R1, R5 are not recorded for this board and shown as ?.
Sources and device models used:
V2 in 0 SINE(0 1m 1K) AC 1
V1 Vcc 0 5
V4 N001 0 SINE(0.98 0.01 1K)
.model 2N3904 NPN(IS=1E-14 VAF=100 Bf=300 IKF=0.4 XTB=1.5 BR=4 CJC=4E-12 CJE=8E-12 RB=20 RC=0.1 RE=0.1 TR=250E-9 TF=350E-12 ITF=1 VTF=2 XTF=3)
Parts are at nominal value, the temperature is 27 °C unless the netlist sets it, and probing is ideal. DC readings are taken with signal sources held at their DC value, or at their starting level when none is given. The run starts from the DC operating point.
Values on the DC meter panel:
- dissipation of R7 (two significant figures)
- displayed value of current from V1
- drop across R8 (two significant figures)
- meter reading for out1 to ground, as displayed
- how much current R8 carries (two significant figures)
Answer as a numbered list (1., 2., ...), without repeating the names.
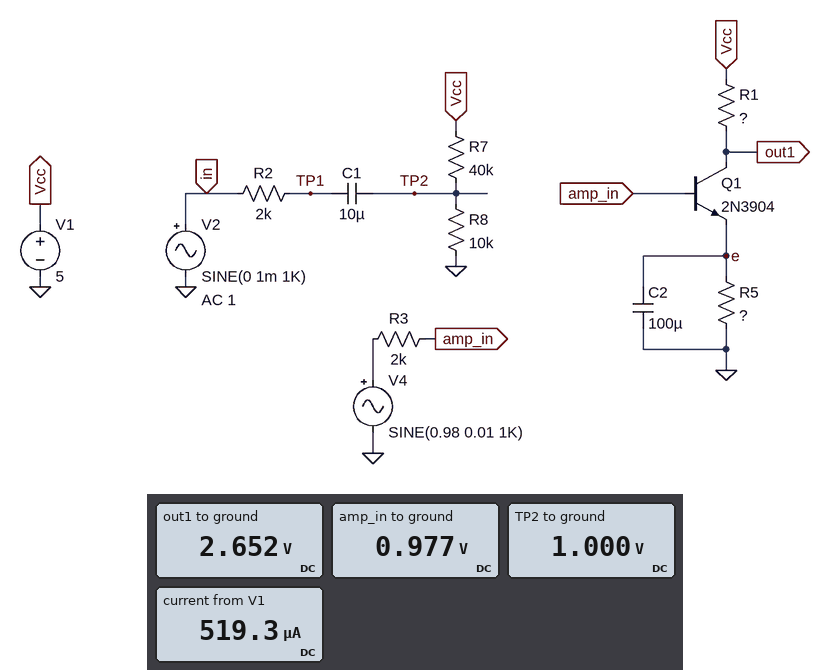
1. 400 µW
2. 519.3 µA
3. 1.0 V
4. 2.652 V
5. 100 µA
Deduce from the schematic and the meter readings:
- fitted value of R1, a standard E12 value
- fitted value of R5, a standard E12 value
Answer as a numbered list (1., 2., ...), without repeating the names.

1. 5.6 kΩ
2. 820 Ω
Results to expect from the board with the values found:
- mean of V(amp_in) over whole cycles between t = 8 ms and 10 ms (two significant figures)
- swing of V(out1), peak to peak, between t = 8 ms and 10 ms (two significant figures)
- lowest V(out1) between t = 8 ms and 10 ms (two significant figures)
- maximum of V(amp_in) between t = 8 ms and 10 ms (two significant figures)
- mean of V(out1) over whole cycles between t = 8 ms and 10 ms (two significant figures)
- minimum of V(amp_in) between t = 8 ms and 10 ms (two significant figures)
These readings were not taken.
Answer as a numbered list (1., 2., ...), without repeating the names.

1. 980 mV
2. 1.6 V
3. 1.8 V
4. 990 mV
5. 2.6 V
6. 970 mV
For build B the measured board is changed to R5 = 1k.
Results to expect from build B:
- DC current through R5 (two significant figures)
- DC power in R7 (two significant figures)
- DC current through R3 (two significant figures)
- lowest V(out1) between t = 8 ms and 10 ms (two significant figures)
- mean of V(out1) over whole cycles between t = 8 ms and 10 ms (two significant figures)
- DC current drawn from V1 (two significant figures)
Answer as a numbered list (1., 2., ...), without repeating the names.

1. 350 µA
2. 400 µW
3. 1.1 µA
4. 2.3 V
5. 3.0 V
6. 450 µA
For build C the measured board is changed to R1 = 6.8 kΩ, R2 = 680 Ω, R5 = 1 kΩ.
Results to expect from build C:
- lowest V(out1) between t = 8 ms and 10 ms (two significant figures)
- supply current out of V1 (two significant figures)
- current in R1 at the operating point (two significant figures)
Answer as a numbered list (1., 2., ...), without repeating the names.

1. 1.7 V
2. 450 µA
3. 350 µA
